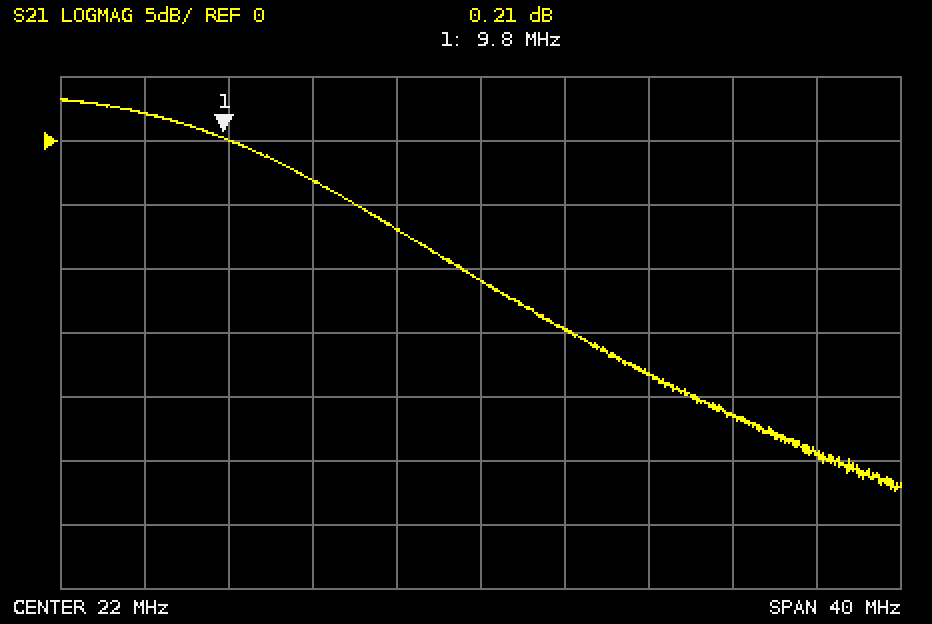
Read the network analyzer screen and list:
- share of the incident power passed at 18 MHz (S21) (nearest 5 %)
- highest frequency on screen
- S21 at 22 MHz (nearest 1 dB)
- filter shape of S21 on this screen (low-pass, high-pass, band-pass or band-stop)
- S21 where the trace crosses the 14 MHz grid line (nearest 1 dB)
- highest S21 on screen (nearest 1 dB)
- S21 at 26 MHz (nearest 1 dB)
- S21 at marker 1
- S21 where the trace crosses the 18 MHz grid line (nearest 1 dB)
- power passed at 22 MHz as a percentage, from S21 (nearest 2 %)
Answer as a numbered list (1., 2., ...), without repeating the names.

1. 20 %
2. 42 MHz
3. -11 dB
4. low-pass
5. -3 dB
6. 3 dB
7. -15 dB
8. 0.21 dB
9. -7 dB
10. 8 %
